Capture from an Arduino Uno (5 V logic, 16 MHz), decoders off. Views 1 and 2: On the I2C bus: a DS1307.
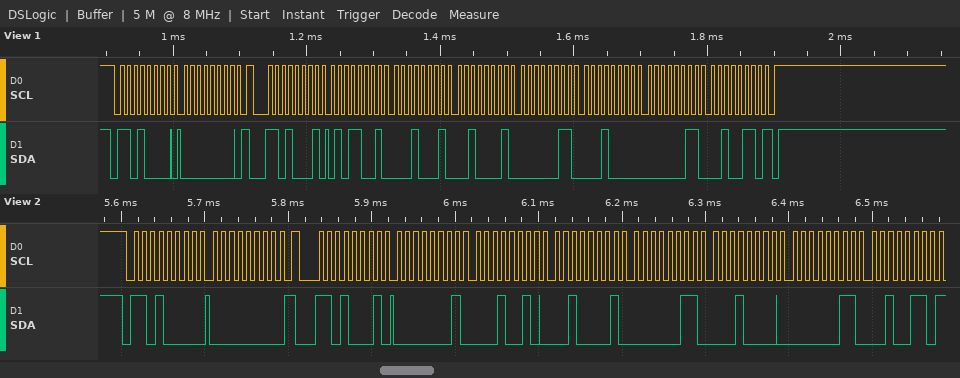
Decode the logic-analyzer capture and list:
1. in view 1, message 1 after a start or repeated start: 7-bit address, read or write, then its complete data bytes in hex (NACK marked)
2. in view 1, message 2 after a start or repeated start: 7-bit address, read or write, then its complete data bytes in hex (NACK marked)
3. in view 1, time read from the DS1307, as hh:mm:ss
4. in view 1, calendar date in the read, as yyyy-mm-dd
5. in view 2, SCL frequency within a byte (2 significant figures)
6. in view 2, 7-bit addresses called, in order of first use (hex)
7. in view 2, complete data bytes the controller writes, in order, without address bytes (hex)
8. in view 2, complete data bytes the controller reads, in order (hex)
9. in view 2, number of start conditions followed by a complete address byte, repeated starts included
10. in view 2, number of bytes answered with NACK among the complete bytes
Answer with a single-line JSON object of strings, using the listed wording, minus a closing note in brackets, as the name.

{"in view 1, message 1 after a start or repeated start: 7-bit address, read or write, then its complete data bytes in hex": "0x68 write: 00", "in view 1, message 2 after a start or repeated start: 7-bit address, read or write, then its complete data bytes in hex": "0x68 read: 59 11 21 03 10 03 26 NACK", "in view 1, time read from the DS1307, as hh:mm:ss": "21:11:59", "in view 1, calendar date in the read, as yyyy-mm-dd": "2026-03-10", "in view 2, SCL frequency within a byte": "100 kHz", "in view 2, 7-bit addresses called, in order of first use": "0x68", "in view 2, complete data bytes the controller writes, in order, without address bytes": "00", "in view 2, complete data bytes the controller reads, in order": "01 12 21 03 10 03 26", "in view 2, number of start conditions followed by a complete address byte, repeated starts included": "2", "in view 2, number of bytes answered with NACK among the complete bytes": "1"}
